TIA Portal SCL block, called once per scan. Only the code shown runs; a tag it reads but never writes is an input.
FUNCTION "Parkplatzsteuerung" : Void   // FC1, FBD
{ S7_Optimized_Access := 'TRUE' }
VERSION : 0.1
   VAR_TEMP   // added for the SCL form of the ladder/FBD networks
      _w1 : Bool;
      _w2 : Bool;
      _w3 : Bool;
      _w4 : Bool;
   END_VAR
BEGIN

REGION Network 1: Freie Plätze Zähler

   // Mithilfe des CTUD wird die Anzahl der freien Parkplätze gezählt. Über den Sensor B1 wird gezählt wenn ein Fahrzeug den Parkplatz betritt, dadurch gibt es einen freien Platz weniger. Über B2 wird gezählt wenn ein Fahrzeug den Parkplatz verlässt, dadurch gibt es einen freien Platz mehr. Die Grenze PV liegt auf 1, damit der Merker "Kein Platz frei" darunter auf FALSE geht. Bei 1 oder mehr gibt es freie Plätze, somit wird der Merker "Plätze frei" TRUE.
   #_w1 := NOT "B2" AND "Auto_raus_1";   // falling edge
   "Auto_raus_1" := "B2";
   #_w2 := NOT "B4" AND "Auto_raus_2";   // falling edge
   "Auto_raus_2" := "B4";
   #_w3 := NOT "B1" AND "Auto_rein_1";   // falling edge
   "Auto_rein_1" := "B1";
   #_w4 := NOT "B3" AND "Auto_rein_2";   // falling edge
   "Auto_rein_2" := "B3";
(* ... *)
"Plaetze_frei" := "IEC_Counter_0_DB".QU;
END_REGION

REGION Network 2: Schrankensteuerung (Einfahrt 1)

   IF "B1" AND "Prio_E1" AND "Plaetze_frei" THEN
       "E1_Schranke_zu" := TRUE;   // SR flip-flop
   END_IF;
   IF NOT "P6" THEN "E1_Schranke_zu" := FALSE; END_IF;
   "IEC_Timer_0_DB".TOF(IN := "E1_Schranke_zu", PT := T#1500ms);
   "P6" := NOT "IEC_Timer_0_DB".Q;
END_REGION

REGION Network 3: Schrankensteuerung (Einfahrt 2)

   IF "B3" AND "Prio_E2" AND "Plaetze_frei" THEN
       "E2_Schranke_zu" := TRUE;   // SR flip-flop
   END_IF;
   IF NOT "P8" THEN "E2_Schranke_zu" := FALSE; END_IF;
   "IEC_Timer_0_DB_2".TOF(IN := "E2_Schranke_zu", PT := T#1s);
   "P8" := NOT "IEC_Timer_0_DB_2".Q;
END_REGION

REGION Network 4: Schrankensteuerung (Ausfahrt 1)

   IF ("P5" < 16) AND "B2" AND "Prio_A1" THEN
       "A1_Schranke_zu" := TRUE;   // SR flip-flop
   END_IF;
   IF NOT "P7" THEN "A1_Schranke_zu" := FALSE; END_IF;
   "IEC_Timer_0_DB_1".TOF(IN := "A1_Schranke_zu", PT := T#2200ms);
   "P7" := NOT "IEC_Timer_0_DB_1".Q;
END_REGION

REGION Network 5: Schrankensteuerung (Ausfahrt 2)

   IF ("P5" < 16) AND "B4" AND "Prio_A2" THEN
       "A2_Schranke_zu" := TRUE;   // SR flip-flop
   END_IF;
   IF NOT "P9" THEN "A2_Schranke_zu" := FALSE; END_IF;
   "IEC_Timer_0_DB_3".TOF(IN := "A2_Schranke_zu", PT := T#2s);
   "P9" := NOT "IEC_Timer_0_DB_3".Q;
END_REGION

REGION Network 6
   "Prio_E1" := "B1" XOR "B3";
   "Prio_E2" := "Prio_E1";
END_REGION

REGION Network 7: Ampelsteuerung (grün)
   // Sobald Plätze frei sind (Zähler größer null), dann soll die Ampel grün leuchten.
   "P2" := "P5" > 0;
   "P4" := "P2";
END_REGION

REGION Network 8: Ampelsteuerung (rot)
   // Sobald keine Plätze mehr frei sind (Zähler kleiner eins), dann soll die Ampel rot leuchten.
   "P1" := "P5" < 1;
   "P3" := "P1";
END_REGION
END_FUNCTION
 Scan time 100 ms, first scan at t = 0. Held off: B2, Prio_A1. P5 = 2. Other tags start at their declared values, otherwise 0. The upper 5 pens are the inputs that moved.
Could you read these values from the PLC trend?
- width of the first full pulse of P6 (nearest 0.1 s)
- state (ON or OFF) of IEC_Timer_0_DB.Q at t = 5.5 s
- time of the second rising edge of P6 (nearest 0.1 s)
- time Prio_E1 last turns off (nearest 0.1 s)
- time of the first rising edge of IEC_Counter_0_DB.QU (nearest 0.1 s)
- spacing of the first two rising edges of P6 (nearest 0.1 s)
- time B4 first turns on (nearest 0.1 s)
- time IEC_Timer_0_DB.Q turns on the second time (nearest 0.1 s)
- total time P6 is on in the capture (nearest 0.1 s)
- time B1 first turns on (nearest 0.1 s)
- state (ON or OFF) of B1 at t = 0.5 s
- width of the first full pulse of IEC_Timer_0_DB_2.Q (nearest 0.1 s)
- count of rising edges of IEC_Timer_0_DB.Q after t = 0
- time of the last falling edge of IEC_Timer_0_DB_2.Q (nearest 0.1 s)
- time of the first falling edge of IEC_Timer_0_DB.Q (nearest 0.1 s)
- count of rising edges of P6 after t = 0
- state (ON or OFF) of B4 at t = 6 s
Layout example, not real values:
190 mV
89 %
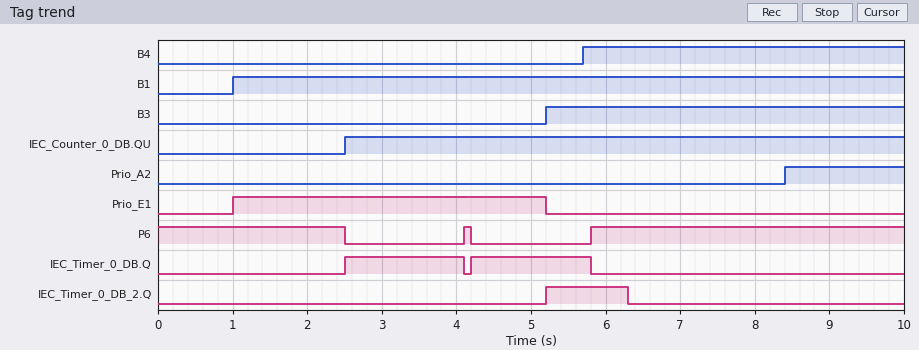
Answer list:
0.1 s
ON
5.8 s
5.2 s
2.5 s
1.7 s
5.7 s
4.2 s
6.8 s
1.0 s
OFF
1.1 s
2
6.3 s
4.1 s
2
ON
